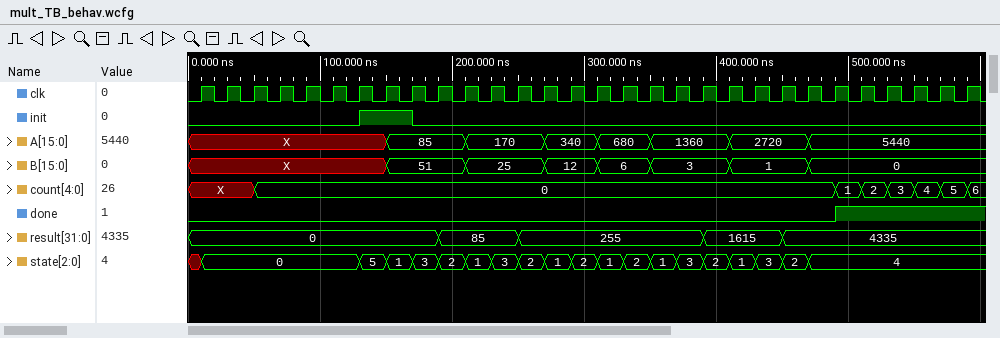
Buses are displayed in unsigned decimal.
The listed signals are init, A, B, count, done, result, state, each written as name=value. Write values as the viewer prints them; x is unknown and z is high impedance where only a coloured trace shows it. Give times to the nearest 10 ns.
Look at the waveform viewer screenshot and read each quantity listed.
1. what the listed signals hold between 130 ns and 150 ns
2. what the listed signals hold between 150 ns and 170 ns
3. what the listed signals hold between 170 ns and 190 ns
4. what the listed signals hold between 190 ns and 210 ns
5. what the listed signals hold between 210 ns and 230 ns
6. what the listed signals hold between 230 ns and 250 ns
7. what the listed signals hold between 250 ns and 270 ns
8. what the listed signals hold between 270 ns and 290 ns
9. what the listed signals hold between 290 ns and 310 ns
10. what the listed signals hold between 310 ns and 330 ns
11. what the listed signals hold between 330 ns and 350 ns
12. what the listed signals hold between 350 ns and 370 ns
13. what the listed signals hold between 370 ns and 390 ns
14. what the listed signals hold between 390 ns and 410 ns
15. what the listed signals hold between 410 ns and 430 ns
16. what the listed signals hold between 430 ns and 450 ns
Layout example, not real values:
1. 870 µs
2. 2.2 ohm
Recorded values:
1. init=1, A=X, B=X, count=0, done=0, result=0, state=5
2. init=1, A=85, B=51, count=0, done=0, result=0, state=1
3. init=0, A=85, B=51, count=0, done=0, result=0, state=3
4. init=0, A=85, B=51, count=0, done=0, result=85, state=2
5. init=0, A=170, B=25, count=0, done=0, result=85, state=1
6. init=0, A=170, B=25, count=0, done=0, result=85, state=3
7. init=0, A=170, B=25, count=0, done=0, result=255, state=2
8. init=0, A=340, B=12, count=0, done=0, result=255, state=1
9. init=0, A=340, B=12, count=0, done=0, result=255, state=2
10. init=0, A=680, B=6, count=0, done=0, result=255, state=1
11. init=0, A=680, B=6, count=0, done=0, result=255, state=2
12. init=0, A=1360, B=3, count=0, done=0, result=255, state=1
13. init=0, A=1360, B=3, count=0, done=0, result=255, state=3
14. init=0, A=1360, B=3, count=0, done=0, result=1615, state=2
15. init=0, A=2720, B=1, count=0, done=0, result=1615, state=1
16. init=0, A=2720, B=1, count=0, done=0, result=1615, state=3
